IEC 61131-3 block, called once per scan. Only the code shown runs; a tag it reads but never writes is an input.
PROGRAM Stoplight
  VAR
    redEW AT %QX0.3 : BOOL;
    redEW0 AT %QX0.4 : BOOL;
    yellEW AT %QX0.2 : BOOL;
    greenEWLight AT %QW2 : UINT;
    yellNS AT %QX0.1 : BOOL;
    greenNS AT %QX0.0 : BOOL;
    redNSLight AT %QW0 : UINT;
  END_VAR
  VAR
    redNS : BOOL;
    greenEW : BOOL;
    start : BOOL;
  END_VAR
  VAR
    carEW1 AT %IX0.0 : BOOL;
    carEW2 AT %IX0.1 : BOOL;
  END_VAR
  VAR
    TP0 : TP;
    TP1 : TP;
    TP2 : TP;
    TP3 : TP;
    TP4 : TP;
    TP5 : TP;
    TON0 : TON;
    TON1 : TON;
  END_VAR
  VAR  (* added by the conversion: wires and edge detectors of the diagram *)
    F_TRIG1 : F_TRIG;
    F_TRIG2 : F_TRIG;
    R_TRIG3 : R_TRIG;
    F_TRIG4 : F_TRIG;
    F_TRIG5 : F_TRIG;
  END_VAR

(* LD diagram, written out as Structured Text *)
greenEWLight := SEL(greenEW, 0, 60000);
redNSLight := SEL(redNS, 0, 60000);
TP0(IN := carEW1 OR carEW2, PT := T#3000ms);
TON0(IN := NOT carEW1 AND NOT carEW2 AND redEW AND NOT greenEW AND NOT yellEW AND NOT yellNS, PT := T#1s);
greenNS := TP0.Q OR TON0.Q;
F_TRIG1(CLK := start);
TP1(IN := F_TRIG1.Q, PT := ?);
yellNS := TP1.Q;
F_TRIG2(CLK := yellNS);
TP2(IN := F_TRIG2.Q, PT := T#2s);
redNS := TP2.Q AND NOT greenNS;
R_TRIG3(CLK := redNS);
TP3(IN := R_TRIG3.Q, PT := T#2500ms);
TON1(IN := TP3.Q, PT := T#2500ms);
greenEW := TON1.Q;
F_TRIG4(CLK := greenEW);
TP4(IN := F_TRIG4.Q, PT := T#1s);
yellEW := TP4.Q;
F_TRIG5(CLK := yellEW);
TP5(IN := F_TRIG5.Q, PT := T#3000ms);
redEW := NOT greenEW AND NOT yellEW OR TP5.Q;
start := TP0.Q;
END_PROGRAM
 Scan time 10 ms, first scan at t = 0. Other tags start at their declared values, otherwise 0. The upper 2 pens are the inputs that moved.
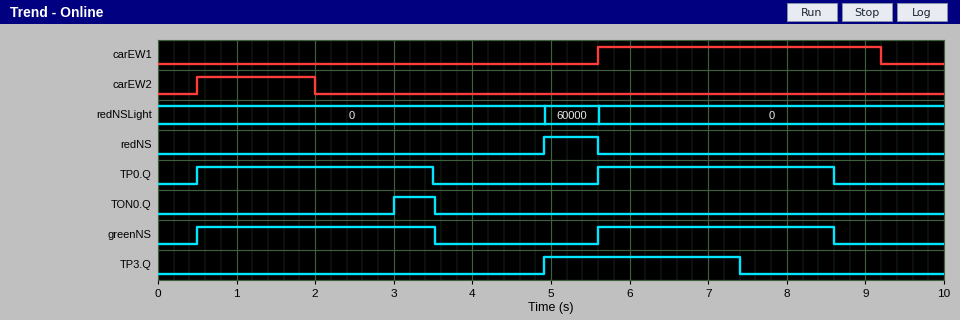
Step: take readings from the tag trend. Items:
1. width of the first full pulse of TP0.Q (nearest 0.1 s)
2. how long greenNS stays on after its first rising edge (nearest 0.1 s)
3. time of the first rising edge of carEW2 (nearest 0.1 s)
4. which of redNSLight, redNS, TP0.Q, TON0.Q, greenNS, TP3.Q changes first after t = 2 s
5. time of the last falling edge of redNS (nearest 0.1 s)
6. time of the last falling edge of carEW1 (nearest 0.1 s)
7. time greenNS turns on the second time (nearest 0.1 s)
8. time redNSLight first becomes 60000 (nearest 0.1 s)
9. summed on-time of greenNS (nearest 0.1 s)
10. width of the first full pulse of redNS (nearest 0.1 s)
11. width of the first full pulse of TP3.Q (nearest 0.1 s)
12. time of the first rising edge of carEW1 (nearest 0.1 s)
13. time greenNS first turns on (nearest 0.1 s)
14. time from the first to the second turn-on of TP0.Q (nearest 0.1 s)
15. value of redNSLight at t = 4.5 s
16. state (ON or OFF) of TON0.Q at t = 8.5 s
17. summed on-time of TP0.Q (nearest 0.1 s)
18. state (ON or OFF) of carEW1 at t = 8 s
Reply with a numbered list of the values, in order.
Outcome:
1. 3.0 s
2. 3.0 s
3. 0.5 s
4. TON0.Q
5. 5.6 s
6. 9.2 s
7. 5.6 s
8. 4.9 s
9. 6.0 s
10. 0.7 s
11. 2.5 s
12. 5.6 s
13. 0.5 s
14. 5.1 s
15. 0
16. OFF
17. 6.0 s
18. ON
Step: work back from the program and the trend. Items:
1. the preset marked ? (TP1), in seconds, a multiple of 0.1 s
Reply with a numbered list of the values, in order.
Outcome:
1. 1.4 s
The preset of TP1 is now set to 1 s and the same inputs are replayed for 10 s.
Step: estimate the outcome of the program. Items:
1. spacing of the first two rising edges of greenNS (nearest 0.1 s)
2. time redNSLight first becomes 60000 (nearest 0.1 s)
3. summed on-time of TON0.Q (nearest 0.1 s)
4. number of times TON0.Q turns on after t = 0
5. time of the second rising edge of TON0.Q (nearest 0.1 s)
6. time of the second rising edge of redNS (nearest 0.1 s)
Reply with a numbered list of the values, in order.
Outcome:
1. 5.0 s
2. 4.5 s
3. 0.6 s
4. 2
5. 5.5 s
6. 9.6 s
